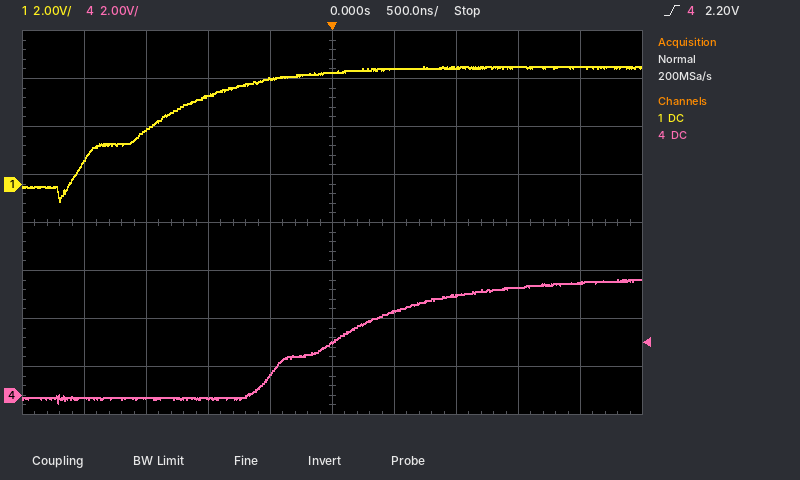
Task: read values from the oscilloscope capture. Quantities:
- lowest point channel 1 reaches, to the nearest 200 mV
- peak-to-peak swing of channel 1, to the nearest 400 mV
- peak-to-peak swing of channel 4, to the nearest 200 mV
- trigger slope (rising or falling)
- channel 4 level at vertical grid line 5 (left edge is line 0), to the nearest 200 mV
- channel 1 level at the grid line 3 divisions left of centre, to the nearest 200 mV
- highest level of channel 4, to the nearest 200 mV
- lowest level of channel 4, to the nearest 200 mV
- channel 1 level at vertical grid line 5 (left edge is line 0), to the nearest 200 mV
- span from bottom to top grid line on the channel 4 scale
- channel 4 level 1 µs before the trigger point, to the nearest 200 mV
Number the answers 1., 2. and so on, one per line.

1. -800 mV
2. 5.6 V
3. 5.2 V
4. rising
5. 2.2 V
6. 2.2 V
7. 4.8 V
8. -400 mV
9. 4.6 V
10. 16 V
11. -200 mV
